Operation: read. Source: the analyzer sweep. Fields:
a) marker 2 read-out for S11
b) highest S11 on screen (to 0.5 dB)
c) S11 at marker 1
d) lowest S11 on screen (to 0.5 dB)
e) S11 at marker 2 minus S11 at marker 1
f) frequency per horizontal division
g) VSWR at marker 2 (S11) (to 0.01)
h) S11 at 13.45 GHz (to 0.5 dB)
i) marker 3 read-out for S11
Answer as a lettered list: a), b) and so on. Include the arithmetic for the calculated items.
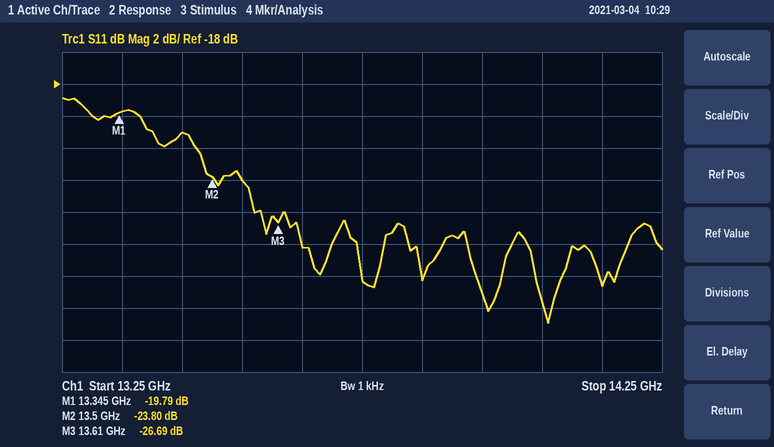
a) -23.80 dB
b) -19.0 dB
c) -19.79 dB
d) -33.0 dB
e) -23.8 − (-19.79) = -4.01 dB
f) 100 MHz
g) (1 + 0.0646)/(1 − 0.0646) ≈ 1.14
h) -21.0 dB
i) -26.69 dB
